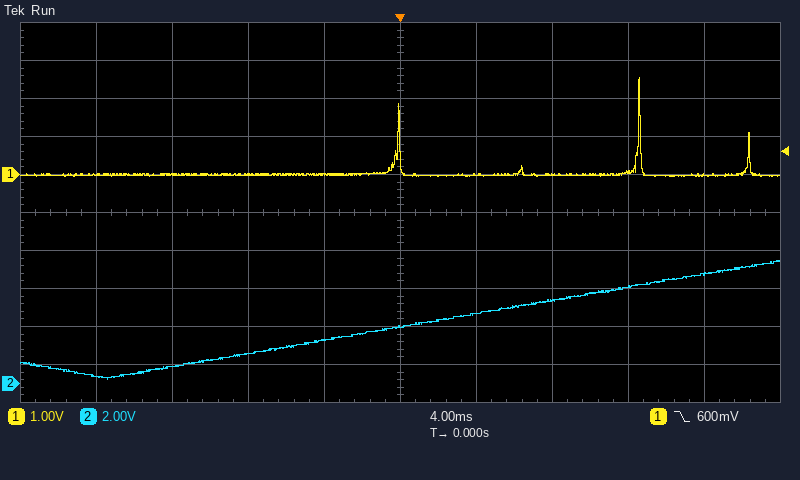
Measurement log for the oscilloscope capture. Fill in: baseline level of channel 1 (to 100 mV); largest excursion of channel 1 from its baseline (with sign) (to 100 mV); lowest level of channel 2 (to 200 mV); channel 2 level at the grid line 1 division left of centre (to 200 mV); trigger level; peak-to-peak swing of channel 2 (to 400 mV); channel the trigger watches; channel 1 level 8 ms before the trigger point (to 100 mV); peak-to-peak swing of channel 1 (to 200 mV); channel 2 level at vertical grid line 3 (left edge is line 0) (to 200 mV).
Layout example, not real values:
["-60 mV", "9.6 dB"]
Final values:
["0.0 V", "+2.6 V", "200 mV", "2.2 V", "600 mV", "6.4 V", "channel 1", "0.0 V", "2.6 V", "1.6 V"]
